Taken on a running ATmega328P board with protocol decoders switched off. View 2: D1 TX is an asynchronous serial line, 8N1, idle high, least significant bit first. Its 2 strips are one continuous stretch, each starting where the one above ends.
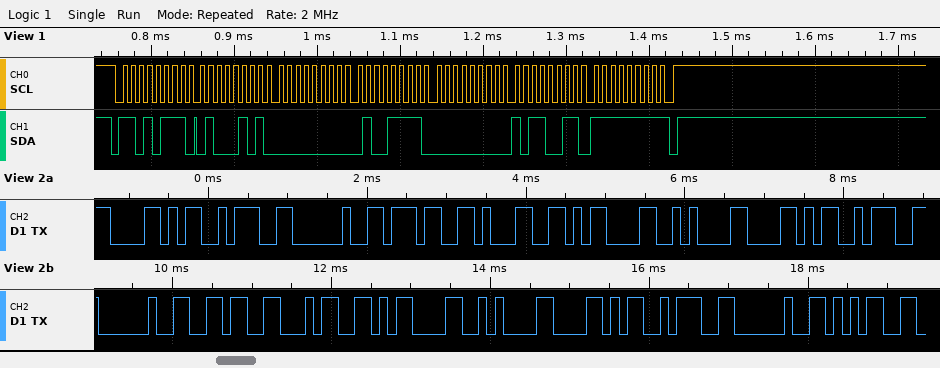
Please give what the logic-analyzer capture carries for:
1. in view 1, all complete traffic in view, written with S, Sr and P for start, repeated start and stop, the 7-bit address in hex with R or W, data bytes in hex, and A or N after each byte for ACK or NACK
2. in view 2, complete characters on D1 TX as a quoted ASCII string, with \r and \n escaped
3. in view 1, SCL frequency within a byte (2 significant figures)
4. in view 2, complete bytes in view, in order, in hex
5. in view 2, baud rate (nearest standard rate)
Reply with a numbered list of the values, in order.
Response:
1. S 6BR A 45 A 00 A 4F A 00 A B3 A FF N P
2. "X: 71\r\nX: 64\r\nX: 5"
3. 100 kHz
4. 58 3A 20 37 31 0D 0A 58 3A 20 36 34 0D 0A 58 3A 20 35
5. 9600 baud
